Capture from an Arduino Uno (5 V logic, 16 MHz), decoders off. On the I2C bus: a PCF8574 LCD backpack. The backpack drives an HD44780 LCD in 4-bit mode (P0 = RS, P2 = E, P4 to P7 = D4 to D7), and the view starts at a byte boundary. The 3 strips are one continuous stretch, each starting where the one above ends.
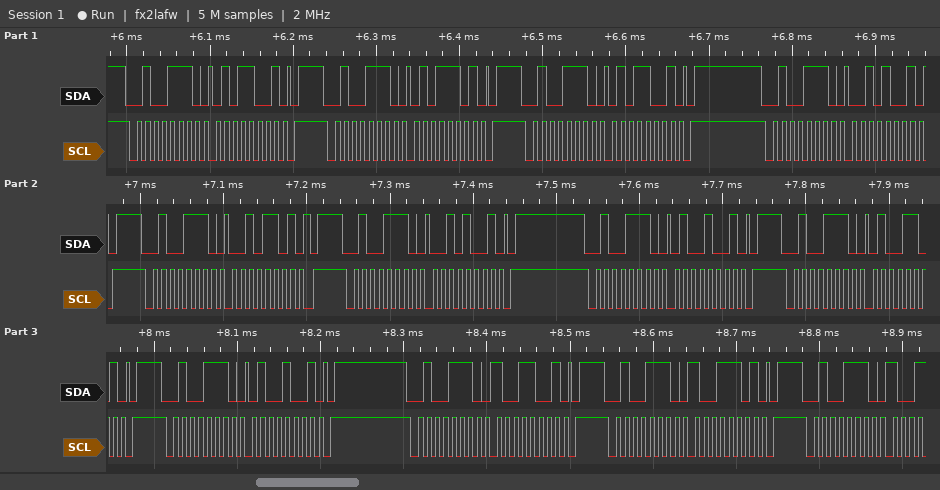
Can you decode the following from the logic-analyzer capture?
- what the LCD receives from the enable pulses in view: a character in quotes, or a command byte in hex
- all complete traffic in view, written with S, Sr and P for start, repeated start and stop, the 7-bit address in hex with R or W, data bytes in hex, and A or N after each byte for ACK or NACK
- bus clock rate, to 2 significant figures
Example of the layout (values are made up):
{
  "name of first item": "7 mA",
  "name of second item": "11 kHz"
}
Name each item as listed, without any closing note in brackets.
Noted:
{
  "what the LCD receives from the enable pulses in view: a character in quotes, or a command byte in hex": "'R'",
  "all complete traffic in view, written with S, Sr and P for start, repeated start and stop, the 7-bit address in hex with R or W, data bytes in hex, and A or N after each byte for ACK or NACK": "S 27W A 59 A P S 27W A 5D A P S 27W A 59 A P S 27W A 29 A P S 27W A 2D A P S 27W A 29 A P S 27W A 49 A P S 27W A 4D A P S 27W A 49 A P S 27W A 99 A P S 27W A 9D A P S 27W A",
  "bus clock rate, to 2 significant figures": "100 kHz"
}
